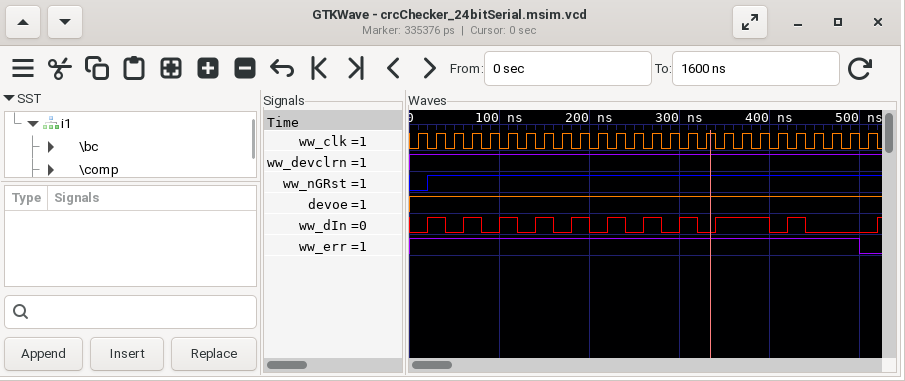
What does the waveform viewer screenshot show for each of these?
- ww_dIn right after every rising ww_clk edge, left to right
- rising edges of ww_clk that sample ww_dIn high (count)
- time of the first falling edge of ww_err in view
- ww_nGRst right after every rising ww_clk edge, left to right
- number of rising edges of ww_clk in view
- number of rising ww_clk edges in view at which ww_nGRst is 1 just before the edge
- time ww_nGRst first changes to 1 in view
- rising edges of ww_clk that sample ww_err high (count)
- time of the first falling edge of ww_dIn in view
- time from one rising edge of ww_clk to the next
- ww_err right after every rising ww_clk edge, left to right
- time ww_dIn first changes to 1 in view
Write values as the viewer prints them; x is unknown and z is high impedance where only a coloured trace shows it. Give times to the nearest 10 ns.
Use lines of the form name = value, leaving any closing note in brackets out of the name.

ww_dIn right after every rising ww_clk edge, left to right = 0 1 0 1 0 1 0 1 0 1 0 1 0 1 0 1 0 1 1 1 0 1 0 0 0 0
rising edges of ww_clk that sample ww_dIn high = 12
time of the first falling edge of ww_err in view = 500 ns
ww_nGRst right after every rising ww_clk edge, left to right = 0 1 1 1 1 1 1 1 1 1 1 1 1 1 1 1 1 1 1 1 1 1 1 1 1 1
number of rising edges of ww_clk in view = 26
number of rising ww_clk edges in view at which ww_nGRst is 1 just before the edge = 25
time ww_nGRst first changes to 1 in view = 20 ns
rising edges of ww_clk that sample ww_err high = 25
time of the first falling edge of ww_dIn in view = 40 ns
time from one rising edge of ww_clk to the next = 20 ns
ww_err right after every rising ww_clk edge, left to right = 1 1 1 1 1 1 1 1 1 1 1 1 1 1 1 1 1 1 1 1 1 1 1 1 1 0
time ww_dIn first changes to 1 in view = 20 ns
